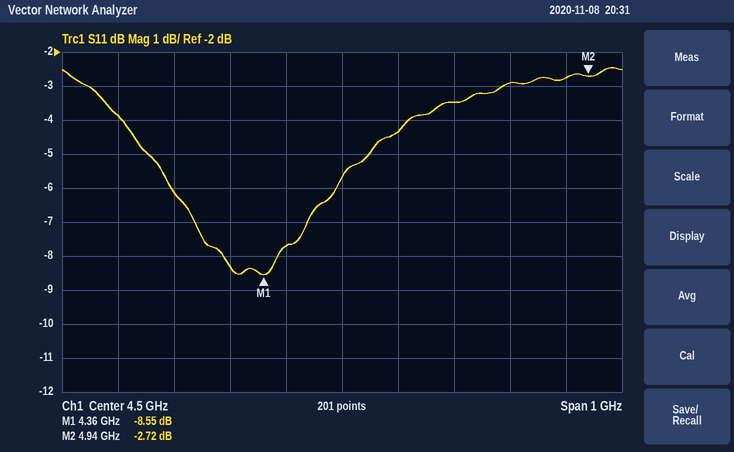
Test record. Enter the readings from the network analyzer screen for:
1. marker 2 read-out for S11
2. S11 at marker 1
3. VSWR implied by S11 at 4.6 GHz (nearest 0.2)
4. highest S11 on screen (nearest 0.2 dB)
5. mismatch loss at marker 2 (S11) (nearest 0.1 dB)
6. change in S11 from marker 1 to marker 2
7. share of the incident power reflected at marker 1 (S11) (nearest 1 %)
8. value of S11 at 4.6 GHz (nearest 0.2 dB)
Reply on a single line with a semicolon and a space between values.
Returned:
-2.72 dB; -8.55 dB; 4.0; -2.4 dB; 3.3 dB; 5.83 dB; 14 %; -4.4 dB
